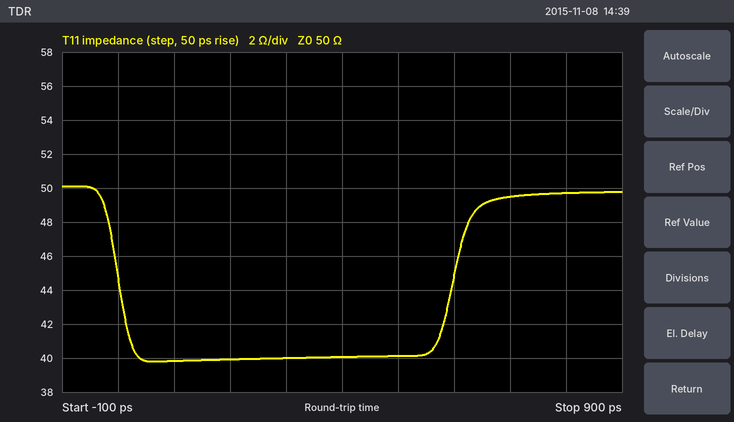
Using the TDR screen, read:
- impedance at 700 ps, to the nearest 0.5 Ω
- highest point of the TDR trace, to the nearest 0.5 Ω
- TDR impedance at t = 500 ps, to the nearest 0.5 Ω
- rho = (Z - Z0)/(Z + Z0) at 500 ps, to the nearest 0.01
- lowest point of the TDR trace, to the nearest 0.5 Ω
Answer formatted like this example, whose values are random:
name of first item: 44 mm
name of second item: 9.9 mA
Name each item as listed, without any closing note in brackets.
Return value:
impedance at 700 ps, to the nearest 0.5 Ω: 49.5 Ω
highest point of the TDR trace, to the nearest 0.5 Ω: 50.0 Ω
TDR impedance at t = 500 ps, to the nearest 0.5 Ω: 40.0 Ω
rho = (Z - Z0)/(Z + Z0) at 500 ps, to the nearest 0.01: -0.11
lowest point of the TDR trace, to the nearest 0.5 Ω: 40.0 Ω
